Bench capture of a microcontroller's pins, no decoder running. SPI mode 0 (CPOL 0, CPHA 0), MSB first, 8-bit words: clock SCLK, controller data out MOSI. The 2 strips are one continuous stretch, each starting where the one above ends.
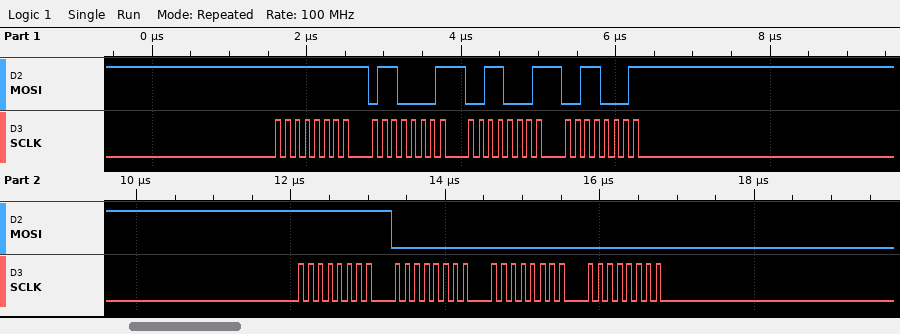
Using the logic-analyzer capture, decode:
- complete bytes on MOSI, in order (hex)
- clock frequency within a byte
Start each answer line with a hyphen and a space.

- FF 61 31 31 FF 00 00 00
- 8 MHz
